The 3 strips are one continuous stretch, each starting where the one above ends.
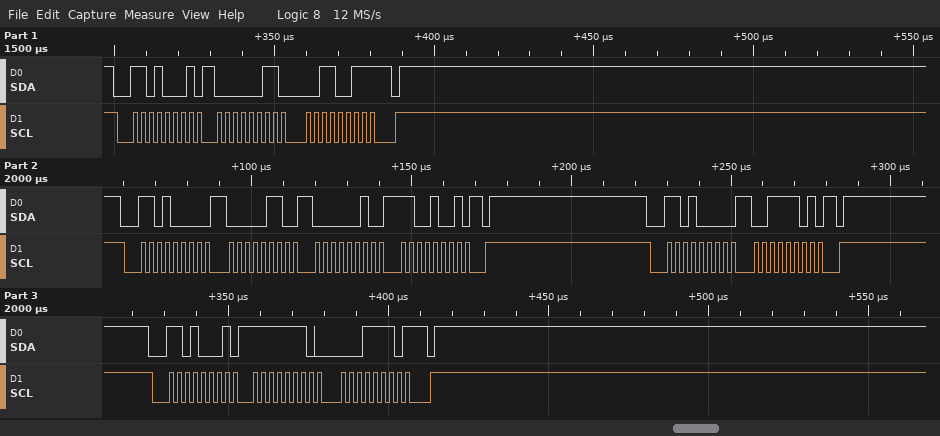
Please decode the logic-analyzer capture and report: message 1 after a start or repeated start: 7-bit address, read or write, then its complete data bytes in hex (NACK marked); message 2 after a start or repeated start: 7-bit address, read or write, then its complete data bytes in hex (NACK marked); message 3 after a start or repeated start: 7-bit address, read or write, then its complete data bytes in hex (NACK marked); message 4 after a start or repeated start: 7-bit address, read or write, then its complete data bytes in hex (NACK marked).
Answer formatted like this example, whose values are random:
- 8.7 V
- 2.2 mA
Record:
- 0x68 read: 03 33 NACK
- 0x68 write: 06 02 C9
- 0x68 write: 3D
- 0x68 read: FE 1E NACK
